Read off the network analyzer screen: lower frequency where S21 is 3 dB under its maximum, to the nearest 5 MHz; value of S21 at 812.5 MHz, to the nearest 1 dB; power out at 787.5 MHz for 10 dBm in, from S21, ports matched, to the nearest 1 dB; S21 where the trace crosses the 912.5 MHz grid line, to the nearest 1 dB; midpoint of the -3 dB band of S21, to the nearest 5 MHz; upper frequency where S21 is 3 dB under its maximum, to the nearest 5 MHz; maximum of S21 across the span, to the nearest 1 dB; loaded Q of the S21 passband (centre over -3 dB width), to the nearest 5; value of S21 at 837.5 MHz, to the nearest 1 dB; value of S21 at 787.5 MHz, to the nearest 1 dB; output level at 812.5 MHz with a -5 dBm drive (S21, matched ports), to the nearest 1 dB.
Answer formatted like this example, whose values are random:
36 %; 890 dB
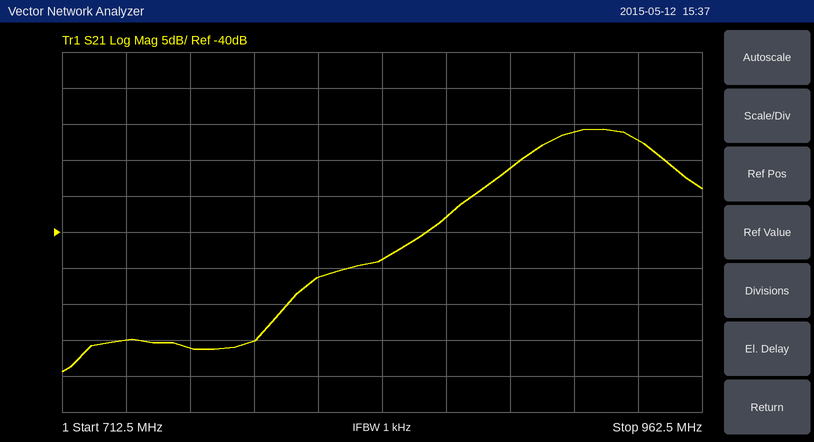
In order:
895 MHz; -46 dB; -45 dBm; -26 dB; 920 MHz; 945 MHz; -26 dB; 20; -44 dB; -55 dB; -51 dBm
